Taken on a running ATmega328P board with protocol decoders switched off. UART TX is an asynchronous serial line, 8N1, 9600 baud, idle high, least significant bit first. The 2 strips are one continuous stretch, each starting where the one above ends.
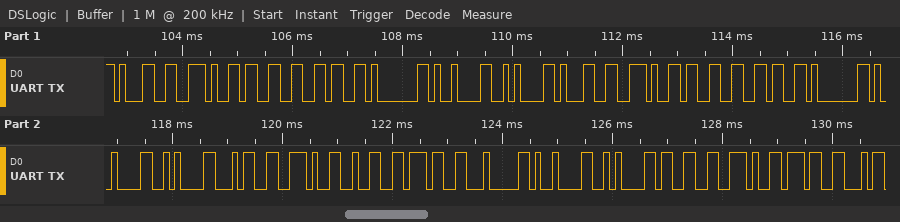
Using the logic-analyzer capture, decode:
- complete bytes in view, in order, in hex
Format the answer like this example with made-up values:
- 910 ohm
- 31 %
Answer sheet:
- 0x31 0x2E 0x33 0x36 0x01 0x09 0x0A 0x31 0x2E 0x33 0x36 0x01 0x09 0x0A 0x34 0x2E 0x32 0x37 0x04 0x09 0x0A 0x33 0x2E 0x37
